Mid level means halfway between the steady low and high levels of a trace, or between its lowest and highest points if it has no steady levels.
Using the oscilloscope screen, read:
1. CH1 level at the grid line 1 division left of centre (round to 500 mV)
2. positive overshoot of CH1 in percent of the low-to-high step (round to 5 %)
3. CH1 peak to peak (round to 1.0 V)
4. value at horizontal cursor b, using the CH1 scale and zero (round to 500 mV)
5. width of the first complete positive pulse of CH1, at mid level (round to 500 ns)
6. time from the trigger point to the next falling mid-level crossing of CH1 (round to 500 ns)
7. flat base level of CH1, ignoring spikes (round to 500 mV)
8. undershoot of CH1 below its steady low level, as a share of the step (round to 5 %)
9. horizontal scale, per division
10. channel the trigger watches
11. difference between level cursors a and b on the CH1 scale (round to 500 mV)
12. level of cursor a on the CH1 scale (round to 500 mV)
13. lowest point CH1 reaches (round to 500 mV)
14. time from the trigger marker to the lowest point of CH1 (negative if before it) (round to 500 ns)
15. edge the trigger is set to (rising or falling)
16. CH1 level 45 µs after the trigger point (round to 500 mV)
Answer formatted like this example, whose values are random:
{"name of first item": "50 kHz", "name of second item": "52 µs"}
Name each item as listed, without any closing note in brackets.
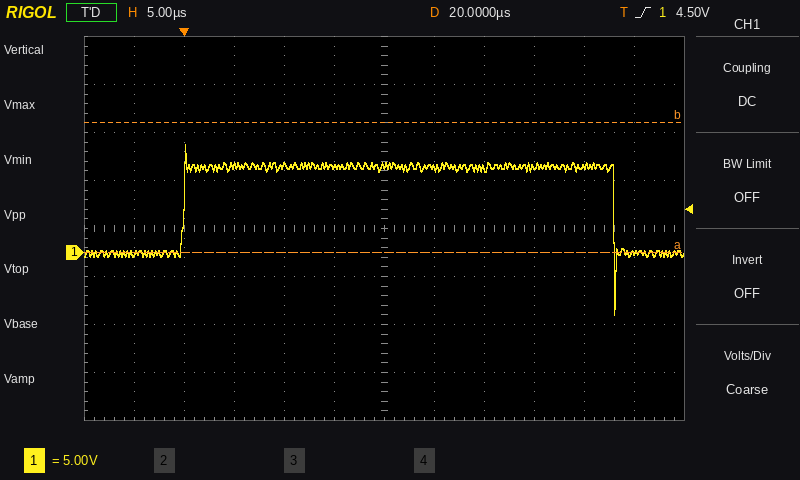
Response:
{"CH1 level at the grid line 1 division left of centre": "9.0 V", "positive overshoot of CH1 in percent of the low-to-high step": "25 %", "CH1 peak to peak": "18.0 V", "value at horizontal cursor b, using the CH1 scale and zero": "13.5 V", "width of the first complete positive pulse of CH1, at mid level": "43.0 µs", "time from the trigger point to the next falling mid-level crossing of CH1": "43.0 µs", "flat base level of CH1, ignoring spikes": "0.0 V", "undershoot of CH1 below its steady low level, as a share of the step": "70 %", "horizontal scale, per division": "5 µs", "channel the trigger watches": "CH1", "difference between level cursors a and b on the CH1 scale": "13.5 V", "level of cursor a on the CH1 scale": "0.0 V", "lowest point CH1 reaches": "-6.5 V", "time from the trigger marker to the lowest point of CH1 (negative if before it)": "+43.0 µs", "edge the trigger is set to": "rising", "CH1 level 45 µs after the trigger point": "0.0 V"}
